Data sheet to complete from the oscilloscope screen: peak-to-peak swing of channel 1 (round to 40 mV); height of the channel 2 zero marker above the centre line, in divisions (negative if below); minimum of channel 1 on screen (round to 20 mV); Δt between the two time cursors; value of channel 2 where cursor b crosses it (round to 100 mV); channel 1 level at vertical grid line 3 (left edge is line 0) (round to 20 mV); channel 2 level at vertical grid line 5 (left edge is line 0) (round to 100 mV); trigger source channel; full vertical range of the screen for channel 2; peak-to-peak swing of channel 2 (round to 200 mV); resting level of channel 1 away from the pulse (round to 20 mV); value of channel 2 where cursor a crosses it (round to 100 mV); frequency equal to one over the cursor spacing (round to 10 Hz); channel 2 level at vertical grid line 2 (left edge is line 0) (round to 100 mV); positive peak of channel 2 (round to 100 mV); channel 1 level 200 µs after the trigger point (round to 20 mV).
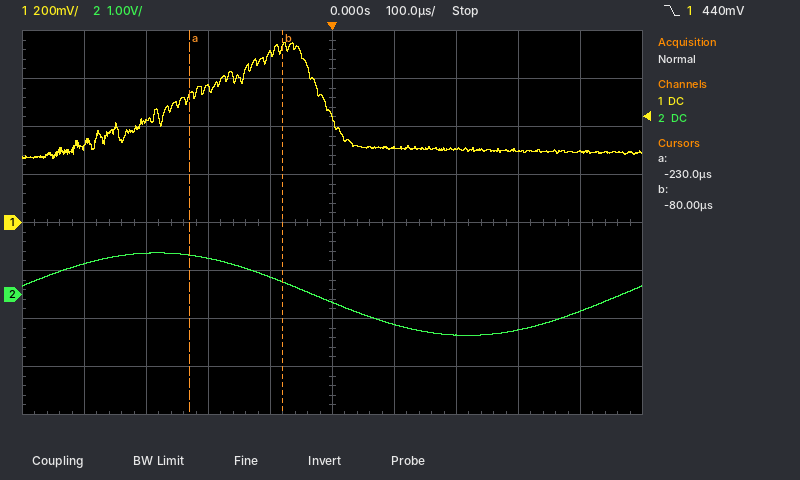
480 mV
-1.5 div
260 mV
150 µs
300 mV
560 mV
-200 mV
channel 1
8 V
1.8 V
300 mV
800 mV
6.67 kHz
900 mV
900 mV
300 mV
